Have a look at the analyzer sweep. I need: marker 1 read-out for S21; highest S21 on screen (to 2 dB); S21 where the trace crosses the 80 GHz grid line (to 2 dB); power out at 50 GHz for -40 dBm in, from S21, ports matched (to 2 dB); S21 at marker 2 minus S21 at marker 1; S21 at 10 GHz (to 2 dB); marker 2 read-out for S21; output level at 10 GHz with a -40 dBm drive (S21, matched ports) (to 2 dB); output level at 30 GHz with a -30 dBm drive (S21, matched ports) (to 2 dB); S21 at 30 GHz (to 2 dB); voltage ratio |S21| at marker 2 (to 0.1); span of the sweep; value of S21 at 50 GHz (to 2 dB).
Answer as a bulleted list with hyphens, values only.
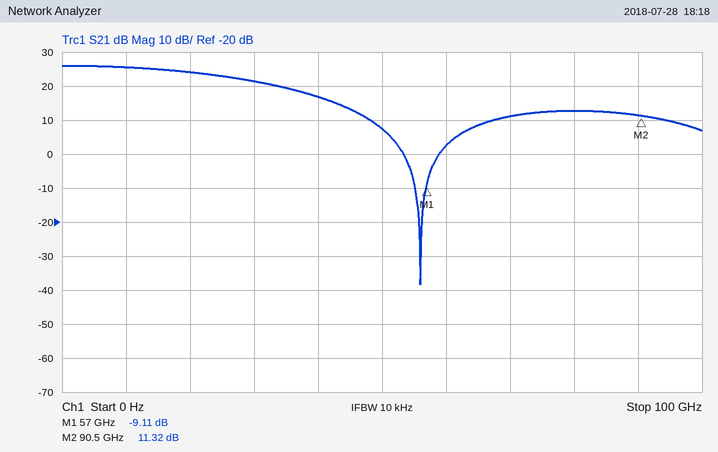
- -9.11 dB
- 26 dB
- 12 dB
- -32 dBm
- 20.43 dB
- 26 dB
- 11.32 dB
- -14 dBm
- -8 dBm
- 22 dB
- 3.7
- 100 GHz
- 8 dB
